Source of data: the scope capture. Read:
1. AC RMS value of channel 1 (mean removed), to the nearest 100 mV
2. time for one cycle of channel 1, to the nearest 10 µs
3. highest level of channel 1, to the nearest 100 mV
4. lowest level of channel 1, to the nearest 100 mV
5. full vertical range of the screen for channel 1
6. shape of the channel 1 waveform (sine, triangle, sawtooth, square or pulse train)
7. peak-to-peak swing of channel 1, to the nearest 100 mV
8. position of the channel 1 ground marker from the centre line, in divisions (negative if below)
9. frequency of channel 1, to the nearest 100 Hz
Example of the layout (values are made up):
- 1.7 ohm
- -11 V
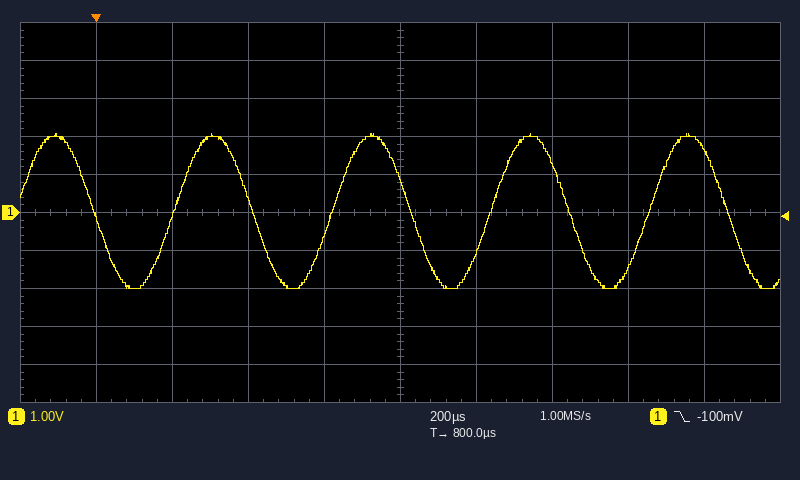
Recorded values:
- 1.4 V
- 420 µs
- 2.1 V
- -2.0 V
- 10 V
- sine
- 4.1 V
- 0.0 div
- 2.4 kHz
